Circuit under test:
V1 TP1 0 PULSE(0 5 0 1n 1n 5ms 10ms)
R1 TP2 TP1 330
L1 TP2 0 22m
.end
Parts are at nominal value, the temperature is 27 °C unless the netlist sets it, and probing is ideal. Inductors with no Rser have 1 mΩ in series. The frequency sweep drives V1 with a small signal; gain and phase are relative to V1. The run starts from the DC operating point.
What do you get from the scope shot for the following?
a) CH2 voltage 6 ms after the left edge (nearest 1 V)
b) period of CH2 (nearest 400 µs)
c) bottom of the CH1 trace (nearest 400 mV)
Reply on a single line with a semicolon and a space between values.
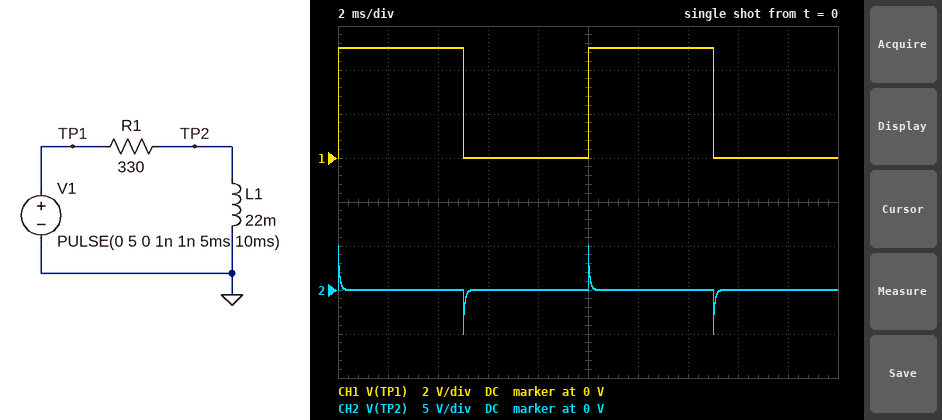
0 V; 10.0 ms; 0 V
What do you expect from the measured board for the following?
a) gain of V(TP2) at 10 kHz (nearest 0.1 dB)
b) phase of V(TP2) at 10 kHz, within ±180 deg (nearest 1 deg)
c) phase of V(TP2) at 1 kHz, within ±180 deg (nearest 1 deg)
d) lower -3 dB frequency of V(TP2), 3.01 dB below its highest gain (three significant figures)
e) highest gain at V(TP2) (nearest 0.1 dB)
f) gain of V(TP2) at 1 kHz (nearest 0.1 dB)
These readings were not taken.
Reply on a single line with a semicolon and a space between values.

-0.2 dB; 13 deg; 67 deg; 2.39 kHz; 0 dB; -8.3 dB
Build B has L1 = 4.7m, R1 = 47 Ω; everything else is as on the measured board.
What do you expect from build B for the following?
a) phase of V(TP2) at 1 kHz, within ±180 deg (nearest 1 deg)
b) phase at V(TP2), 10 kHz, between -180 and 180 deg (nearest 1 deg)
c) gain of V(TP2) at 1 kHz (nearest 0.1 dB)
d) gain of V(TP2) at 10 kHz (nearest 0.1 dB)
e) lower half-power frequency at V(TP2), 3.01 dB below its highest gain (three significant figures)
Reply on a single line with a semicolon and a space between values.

58 deg; 9 deg; -5.5 dB; -0.1 dB; 1.59 kHz
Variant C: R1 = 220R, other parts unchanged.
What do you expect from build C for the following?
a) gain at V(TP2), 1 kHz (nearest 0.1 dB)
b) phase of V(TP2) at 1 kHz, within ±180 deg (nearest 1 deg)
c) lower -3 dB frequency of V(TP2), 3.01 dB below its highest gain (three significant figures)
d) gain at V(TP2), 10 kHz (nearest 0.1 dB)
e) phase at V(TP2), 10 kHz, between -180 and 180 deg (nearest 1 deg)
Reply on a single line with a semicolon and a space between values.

-5.5 dB; 58 deg; 1.59 kHz; -0.1 dB; 9 deg
